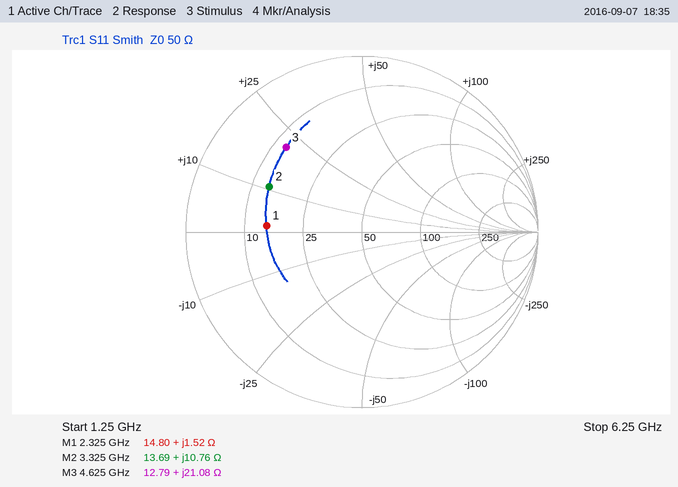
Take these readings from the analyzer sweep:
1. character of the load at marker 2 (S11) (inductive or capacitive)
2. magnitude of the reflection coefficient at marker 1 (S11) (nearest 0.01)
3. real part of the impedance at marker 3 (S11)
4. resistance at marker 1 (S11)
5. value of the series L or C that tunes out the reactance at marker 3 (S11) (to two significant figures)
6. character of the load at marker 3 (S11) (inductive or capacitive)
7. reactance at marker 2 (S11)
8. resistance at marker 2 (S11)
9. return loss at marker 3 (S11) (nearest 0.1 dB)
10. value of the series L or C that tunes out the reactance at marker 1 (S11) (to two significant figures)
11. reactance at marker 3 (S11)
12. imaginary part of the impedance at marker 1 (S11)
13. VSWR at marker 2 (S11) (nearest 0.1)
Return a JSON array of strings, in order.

["inductive", "0.54", "12.79 Ω", "14.80 Ω", "1.6 pF", "inductive", "+10.76 Ω", "13.69 Ω", "3.8 dB", "45 pF", "+21.08 Ω", "+1.52 Ω", "3.8"]
